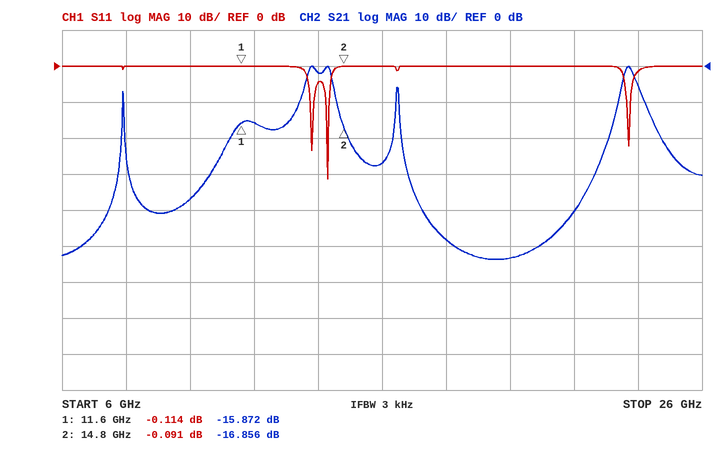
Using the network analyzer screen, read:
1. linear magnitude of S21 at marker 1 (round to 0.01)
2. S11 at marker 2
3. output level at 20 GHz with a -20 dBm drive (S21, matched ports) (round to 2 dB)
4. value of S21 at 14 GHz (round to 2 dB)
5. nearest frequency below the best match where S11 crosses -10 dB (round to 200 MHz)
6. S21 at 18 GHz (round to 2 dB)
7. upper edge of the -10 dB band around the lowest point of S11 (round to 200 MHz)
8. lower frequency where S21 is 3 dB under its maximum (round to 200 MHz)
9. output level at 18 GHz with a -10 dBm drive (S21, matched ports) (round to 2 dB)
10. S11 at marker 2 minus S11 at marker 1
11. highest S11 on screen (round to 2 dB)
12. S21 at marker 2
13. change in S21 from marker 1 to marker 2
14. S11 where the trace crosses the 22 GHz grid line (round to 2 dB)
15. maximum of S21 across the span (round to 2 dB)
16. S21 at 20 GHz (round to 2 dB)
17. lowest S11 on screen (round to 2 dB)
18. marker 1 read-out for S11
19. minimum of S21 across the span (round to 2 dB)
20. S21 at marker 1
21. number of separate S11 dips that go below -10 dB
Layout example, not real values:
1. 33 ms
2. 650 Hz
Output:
1. 0.16
2. -0.091 dB
3. -74 dBm
4. -2 dB
5. 14.2 GHz
6. -48 dB
7. 14.4 GHz
8. 13.6 GHz
9. -58 dBm
10. 0.023 dB
11. 0 dB
12. -16.856 dB
13. -0.984 dB
14. 0 dB
15. 0 dB
16. -54 dB
17. -32 dB
18. -0.114 dB
19. -54 dB
20. -15.872 dB
21. 3
